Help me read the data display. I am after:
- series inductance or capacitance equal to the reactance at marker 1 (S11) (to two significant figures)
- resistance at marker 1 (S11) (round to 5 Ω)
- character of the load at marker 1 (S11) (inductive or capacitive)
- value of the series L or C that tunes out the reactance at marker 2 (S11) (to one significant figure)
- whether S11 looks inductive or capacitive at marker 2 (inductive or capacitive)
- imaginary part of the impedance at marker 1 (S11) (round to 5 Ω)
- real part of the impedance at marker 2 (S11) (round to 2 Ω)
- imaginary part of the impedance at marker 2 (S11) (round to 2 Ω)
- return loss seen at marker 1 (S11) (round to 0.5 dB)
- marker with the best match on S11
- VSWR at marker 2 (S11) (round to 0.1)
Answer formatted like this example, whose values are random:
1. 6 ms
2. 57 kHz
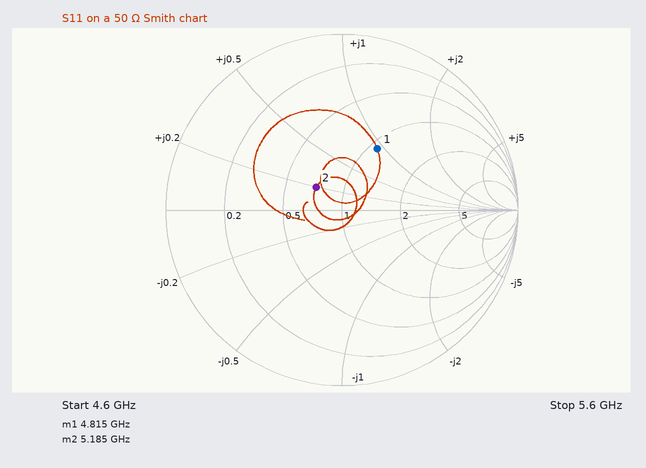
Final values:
1. 1.5 nH
2. 55 Ω
3. inductive
4. 3 pF
5. inductive
6. +45 Ω
7. 36 Ω
8. +10 Ω
9. 8.0 dB
10. marker 2
11. 1.5
